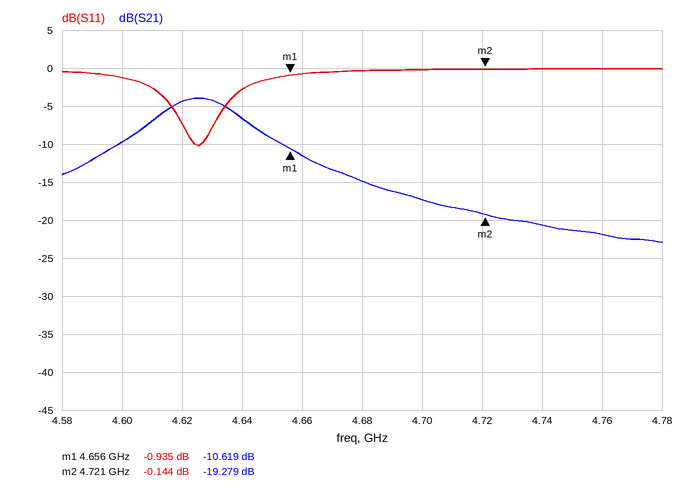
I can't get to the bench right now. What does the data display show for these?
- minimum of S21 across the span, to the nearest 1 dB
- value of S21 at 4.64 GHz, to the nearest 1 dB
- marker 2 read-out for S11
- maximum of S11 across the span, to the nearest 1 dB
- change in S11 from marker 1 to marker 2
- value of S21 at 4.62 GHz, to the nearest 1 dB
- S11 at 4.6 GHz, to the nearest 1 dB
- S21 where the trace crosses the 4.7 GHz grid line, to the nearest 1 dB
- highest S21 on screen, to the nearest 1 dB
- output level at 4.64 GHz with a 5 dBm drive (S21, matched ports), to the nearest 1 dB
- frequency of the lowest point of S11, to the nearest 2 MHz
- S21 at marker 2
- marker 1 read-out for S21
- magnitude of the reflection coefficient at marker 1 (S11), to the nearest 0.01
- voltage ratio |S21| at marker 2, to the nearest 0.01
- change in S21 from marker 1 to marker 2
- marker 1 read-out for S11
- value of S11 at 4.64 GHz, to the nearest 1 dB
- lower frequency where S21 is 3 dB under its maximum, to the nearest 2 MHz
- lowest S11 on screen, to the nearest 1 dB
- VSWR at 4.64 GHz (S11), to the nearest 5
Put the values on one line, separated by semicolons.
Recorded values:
-23 dB; -7 dB; -0.144 dB; 0 dB; 0.791 dB; -4 dB; -1 dB; -17 dB; -4 dB; -2 dBm; 4.626 GHz; -19.279 dB; -10.619 dB; 0.90; 0.11; -8.660 dB; -0.935 dB; -3 dB; 4.610 GHz; -10 dB; 5
